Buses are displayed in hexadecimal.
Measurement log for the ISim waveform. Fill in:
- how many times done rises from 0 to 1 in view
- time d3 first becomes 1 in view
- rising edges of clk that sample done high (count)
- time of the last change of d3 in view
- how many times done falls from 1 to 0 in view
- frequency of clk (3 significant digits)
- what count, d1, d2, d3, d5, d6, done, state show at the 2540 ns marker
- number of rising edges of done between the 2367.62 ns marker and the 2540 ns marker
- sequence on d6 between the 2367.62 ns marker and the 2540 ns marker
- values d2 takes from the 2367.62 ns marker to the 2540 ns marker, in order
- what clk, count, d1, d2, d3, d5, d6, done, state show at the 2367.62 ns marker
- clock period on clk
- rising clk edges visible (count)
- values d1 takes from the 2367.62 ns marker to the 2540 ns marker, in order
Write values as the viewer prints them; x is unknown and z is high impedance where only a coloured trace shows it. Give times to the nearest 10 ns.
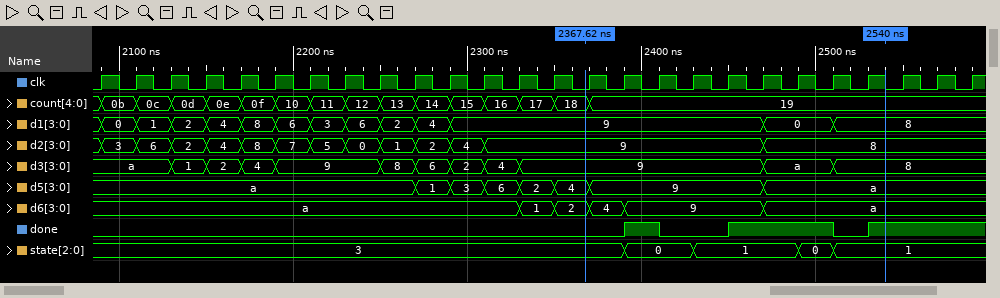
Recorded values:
3
2130 ns
7
2510 ns
2
50.0 MHz
count=19, d1=8, d2=8, d3=8, d5=a, d6=a, done=1, state=1
3
2, 4, 9, a
9, 8
clk=0, count=18, d1=9, d2=9, d3=9, d5=4, d6=2, done=0, state=3
20 ns
26
9, 0, 8
